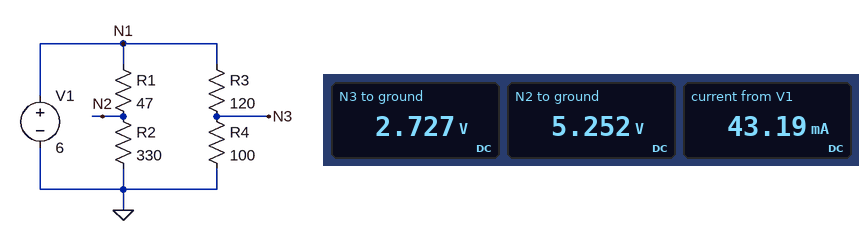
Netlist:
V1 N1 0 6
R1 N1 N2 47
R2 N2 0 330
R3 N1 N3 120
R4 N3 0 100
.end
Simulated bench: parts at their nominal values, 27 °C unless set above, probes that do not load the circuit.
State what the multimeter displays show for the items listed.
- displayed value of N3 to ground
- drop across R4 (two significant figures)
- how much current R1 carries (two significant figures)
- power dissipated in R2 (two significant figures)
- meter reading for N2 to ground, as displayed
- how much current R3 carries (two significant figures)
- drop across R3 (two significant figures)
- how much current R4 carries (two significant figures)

2.727 V
2.7 V
16 mA
84 mW
5.252 V
27 mA
3.3 V
27 mA
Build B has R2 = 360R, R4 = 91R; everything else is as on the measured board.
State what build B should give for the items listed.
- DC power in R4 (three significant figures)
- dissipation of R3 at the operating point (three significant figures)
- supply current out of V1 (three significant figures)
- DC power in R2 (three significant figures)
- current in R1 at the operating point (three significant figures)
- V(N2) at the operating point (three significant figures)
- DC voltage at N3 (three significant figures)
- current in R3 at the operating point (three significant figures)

73.6 mW
97.0 mW
43.2 mA
78.2 mW
14.7 mA
5.31 V
2.59 V
28.4 mA
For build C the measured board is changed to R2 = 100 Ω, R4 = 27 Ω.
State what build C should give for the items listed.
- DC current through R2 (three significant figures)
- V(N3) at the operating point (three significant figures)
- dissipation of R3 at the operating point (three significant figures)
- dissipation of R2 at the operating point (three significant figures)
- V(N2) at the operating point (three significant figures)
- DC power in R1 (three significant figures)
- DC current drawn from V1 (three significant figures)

40.8 mA
1.10 V
200 mW
167 mW
4.08 V
78.3 mW
81.6 mA
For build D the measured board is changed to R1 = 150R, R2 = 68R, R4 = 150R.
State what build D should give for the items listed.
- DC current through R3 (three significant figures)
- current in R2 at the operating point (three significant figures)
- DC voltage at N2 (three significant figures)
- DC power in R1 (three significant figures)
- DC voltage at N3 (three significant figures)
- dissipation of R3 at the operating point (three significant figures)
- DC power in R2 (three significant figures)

22.2 mA
27.5 mA
1.87 V
114 mW
3.33 V
59.3 mW
51.5 mW
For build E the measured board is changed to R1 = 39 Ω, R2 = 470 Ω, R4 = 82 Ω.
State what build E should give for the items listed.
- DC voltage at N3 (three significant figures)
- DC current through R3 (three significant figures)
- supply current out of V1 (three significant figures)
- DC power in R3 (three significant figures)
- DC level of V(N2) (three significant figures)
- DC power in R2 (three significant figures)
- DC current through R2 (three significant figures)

2.44 V
29.7 mA
41.5 mA
106 mW
5.54 V
65.3 mW
11.8 mA
